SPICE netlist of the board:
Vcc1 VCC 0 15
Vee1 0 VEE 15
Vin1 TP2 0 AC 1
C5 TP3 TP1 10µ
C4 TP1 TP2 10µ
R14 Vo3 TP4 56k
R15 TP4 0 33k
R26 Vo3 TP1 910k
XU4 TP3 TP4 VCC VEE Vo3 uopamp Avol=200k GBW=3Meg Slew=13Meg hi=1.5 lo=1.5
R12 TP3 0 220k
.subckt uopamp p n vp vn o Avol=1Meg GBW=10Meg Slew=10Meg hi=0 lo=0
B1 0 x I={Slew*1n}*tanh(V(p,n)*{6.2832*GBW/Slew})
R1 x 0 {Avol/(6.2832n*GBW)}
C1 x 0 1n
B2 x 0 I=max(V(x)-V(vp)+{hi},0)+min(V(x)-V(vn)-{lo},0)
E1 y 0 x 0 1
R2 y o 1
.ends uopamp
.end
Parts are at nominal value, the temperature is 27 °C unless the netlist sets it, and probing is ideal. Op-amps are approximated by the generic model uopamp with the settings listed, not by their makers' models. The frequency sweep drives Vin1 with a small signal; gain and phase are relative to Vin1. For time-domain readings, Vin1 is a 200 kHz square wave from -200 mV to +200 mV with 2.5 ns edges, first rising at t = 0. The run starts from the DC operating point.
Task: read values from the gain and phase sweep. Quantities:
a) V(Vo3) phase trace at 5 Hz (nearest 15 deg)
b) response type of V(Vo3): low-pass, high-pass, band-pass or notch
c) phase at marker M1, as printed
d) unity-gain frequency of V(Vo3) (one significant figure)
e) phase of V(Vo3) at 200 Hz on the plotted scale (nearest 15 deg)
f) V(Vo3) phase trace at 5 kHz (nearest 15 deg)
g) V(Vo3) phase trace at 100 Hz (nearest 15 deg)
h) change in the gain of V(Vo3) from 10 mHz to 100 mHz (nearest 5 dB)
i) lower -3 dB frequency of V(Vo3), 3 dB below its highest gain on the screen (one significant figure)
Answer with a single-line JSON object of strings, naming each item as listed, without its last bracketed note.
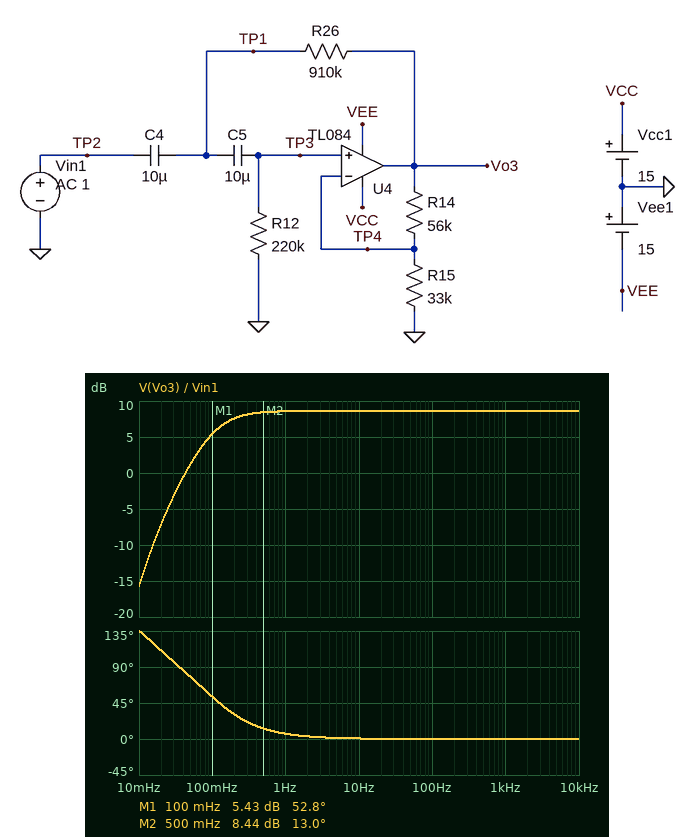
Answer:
{"V(Vo3) phase trace at 5 Hz": "0 deg", "response type of V(Vo3): low-pass, high-pass, band-pass or notch": "high-pass", "phase at marker M1, as printed": "52.8 deg", "unity-gain frequency of V(Vo3)": "40 mHz", "phase of V(Vo3) at 200 Hz on the plotted scale": "0 deg", "V(Vo3) phase trace at 5 kHz": "0 deg", "V(Vo3) phase trace at 100 Hz": "0 deg", "change in the gain of V(Vo3) from 10 mHz to 100 mHz": "20 dB", "lower -3 dB frequency of V(Vo3), 3 dB below its highest gain on the screen": "100 mHz"}
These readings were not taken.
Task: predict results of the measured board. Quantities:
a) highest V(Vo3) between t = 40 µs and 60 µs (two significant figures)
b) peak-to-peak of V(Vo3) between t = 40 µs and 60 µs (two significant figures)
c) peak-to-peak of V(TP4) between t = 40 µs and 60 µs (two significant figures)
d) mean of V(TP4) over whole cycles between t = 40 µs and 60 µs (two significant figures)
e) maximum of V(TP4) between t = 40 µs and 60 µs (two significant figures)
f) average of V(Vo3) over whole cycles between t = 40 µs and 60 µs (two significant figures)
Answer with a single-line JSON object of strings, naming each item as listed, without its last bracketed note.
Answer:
{"highest V(Vo3) between t = 40 µs and 60 µs": "1.1 V", "peak-to-peak of V(Vo3) between t = 40 µs and 60 µs": "1.1 V", "peak-to-peak of V(TP4) between t = 40 µs and 60 µs": "400 mV", "mean of V(TP4) over whole cycles between t = 40 µs and 60 µs": "200 mV", "maximum of V(TP4) between t = 40 µs and 60 µs": "400 mV", "average of V(Vo3) over whole cycles between t = 40 µs and 60 µs": "540 mV"}
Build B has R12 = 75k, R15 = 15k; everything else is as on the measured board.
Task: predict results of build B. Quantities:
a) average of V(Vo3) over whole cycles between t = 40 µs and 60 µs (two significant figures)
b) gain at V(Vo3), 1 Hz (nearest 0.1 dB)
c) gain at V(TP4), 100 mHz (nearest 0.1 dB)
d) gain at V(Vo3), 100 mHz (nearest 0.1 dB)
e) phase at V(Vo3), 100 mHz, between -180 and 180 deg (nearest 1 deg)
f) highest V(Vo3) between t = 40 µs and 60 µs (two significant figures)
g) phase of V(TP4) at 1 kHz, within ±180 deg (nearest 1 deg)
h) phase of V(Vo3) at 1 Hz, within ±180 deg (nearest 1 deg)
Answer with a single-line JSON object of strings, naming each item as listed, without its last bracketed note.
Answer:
{"average of V(Vo3) over whole cycles between t = 40 µs and 60 µs": "950 mV", "gain at V(Vo3), 1 Hz": "13.0 dB", "gain at V(TP4), 100 mHz": "-11.2 dB", "gain at V(Vo3), 100 mHz": "2.3 dB", "phase at V(Vo3), 100 mHz, between -180 and 180 deg": "80 deg", "highest V(Vo3) between t = 40 µs and 60 µs": "1.9 V", "phase of V(TP4) at 1 kHz, within ±180 deg": "0 deg", "phase of V(Vo3) at 1 Hz, within ±180 deg": "20 deg"}
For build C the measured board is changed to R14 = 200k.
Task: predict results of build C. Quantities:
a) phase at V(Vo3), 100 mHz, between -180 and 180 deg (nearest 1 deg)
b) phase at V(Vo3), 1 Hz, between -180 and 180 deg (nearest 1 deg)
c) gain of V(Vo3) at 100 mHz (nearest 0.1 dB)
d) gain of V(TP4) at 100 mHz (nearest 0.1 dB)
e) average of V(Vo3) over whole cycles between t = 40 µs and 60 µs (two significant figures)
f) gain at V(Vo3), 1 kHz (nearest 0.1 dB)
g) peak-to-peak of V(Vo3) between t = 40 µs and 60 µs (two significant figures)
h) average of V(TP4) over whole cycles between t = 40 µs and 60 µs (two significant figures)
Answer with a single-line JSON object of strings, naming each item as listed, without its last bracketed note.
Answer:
{"phase at V(Vo3), 100 mHz, between -180 and 180 deg": "24 deg", "phase at V(Vo3), 1 Hz, between -180 and 180 deg": "2 deg", "gain of V(Vo3) at 100 mHz": "17.4 dB", "gain of V(TP4) at 100 mHz": "0.4 dB", "average of V(Vo3) over whole cycles between t = 40 µs and 60 µs": "1.4 V", "gain at V(Vo3), 1 kHz": "17.0 dB", "peak-to-peak of V(Vo3) between t = 40 µs and 60 µs": "2.8 V", "average of V(TP4) over whole cycles between t = 40 µs and 60 µs": "200 mV"}
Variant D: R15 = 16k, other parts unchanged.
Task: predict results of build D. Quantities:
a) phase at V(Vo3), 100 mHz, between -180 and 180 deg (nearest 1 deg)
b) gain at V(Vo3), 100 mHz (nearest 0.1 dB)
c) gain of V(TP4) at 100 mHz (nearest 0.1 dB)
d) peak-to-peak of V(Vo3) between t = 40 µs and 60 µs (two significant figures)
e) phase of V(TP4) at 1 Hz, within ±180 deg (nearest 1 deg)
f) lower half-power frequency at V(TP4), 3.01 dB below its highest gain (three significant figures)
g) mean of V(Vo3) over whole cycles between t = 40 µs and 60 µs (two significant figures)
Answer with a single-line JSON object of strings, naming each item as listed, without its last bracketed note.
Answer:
{"phase at V(Vo3), 100 mHz, between -180 and 180 deg": "44 deg", "gain at V(Vo3), 100 mHz": "11.4 dB", "gain of V(TP4) at 100 mHz": "-1.6 dB", "peak-to-peak of V(Vo3) between t = 40 µs and 60 µs": "1.8 V", "phase of V(TP4) at 1 Hz, within ±180 deg": "5 deg", "lower half-power frequency at V(TP4), 3.01 dB below its highest gain": "69.1 mHz", "mean of V(Vo3) over whole cycles between t = 40 µs and 60 µs": "900 mV"}
